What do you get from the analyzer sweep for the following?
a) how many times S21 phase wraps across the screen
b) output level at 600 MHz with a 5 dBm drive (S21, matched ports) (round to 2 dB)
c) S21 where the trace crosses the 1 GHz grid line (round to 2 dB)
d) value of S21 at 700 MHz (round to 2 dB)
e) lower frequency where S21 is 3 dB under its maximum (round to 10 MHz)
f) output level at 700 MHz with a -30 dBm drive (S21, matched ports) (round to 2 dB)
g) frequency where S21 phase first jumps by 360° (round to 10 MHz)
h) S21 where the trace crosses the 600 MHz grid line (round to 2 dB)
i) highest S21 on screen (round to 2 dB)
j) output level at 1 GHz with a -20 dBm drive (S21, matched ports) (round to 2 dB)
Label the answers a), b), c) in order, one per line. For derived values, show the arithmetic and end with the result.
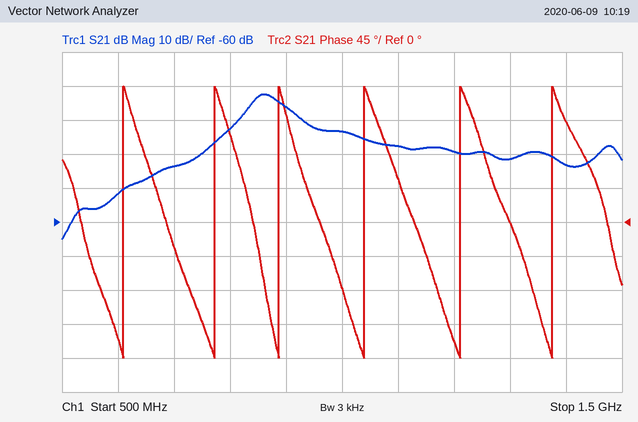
a) 6
b) 5 dBm + (-52 dB) = -46 dBm
c) -34 dB
d) -44 dB
e) 840 MHz
f) -30 dBm + (-44 dB) = -74 dBm
g) 610 MHz
h) -52 dB
i) -22 dB
j) -20 dBm + (-34 dB) = -54 dBm
